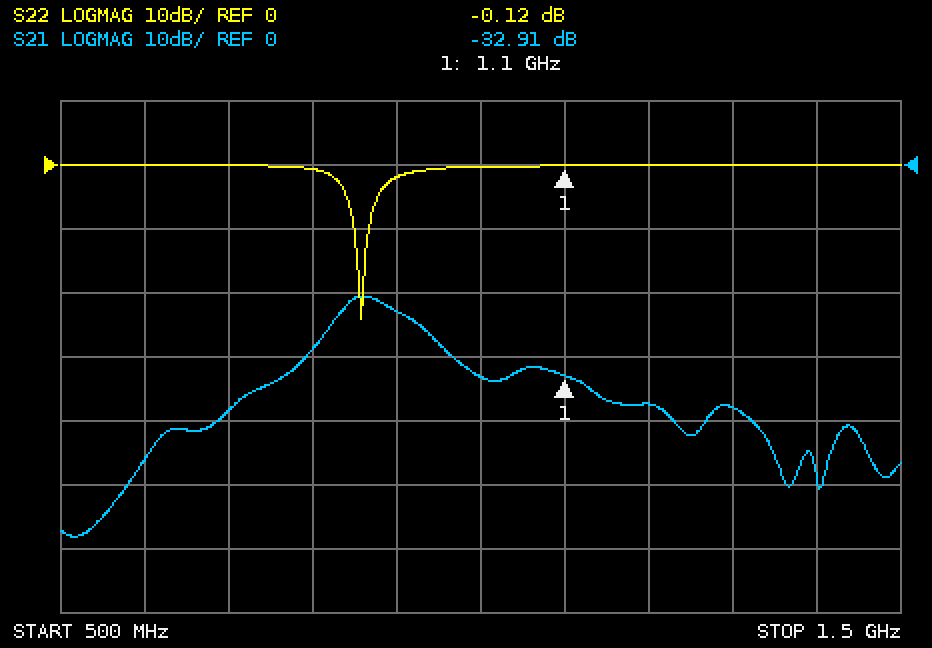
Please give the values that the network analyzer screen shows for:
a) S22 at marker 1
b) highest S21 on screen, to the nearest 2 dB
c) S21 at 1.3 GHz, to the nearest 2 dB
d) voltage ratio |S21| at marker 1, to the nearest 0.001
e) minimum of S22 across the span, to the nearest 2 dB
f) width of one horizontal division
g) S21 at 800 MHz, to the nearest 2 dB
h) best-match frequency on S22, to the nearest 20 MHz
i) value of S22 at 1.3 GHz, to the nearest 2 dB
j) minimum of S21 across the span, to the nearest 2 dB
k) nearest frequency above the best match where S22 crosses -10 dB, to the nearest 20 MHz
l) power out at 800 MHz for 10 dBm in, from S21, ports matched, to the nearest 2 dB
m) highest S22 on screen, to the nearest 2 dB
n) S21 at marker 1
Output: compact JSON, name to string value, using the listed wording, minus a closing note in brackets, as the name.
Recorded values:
{"S22 at marker 1": "-0.12 dB", "highest S21 on screen, to the nearest 2 dB": "-20 dB", "S21 at 1.3 GHz, to the nearest 2 dB": "-38 dB", "voltage ratio |S21| at marker 1, to the nearest 0.001": "0.023", "minimum of S22 across the span, to the nearest 2 dB": "-24 dB", "width of one horizontal division": "100 MHz", "S21 at 800 MHz, to the nearest 2 dB": "-28 dB", "best-match frequency on S22, to the nearest 20 MHz": "860 MHz", "value of S22 at 1.3 GHz, to the nearest 2 dB": "0 dB", "minimum of S21 across the span, to the nearest 2 dB": "-58 dB", "nearest frequency above the best match where S22 crosses -10 dB, to the nearest 20 MHz": "860 MHz", "power out at 800 MHz for 10 dBm in, from S21, ports matched, to the nearest 2 dB": "-18 dBm", "highest S22 on screen, to the nearest 2 dB": "0 dB", "S21 at marker 1": "-32.91 dB"}
